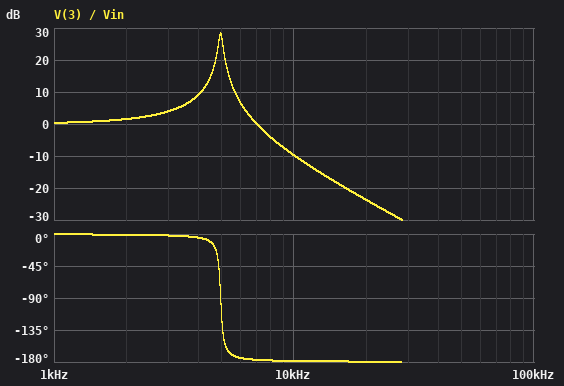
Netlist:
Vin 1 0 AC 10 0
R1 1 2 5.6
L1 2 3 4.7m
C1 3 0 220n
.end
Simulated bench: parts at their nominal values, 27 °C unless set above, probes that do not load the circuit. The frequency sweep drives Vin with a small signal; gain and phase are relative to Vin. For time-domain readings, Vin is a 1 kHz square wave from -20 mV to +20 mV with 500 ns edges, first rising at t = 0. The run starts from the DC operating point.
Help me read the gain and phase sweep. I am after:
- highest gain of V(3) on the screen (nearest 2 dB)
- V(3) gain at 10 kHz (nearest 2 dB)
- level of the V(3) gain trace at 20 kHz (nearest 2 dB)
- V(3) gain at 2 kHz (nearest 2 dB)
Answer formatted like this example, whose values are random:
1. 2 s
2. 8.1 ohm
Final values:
1. 28 dB
2. -10 dB
3. -24 dB
4. 2 dB
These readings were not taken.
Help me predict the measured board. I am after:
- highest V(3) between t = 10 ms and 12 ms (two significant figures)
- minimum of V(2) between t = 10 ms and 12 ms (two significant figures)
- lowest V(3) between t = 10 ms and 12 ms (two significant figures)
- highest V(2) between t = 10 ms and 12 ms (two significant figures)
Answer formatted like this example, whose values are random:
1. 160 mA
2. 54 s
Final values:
1. 150 mV
2. -25 mV
3. -150 mV
4. 25 mV
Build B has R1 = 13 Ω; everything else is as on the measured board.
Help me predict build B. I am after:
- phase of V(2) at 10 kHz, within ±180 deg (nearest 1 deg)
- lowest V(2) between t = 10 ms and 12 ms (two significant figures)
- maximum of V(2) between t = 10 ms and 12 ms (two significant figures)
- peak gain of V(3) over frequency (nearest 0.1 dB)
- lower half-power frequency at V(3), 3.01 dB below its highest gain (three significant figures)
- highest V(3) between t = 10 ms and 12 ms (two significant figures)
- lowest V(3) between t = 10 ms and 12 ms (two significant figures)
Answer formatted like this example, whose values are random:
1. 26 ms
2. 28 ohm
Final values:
1. 3 deg
2. -26 mV
3. 26 mV
4. 21.0 dB
5. 4.71 kHz
6. 87 mV
7. -87 mV
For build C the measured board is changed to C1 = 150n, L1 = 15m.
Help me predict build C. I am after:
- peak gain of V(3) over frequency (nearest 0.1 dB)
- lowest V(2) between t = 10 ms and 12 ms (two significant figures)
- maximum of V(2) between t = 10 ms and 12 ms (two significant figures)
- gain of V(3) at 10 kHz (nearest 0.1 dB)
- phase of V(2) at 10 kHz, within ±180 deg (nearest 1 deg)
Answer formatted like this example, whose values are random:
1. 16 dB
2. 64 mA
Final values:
1. 35.0 dB
2. -21 mV
3. 21 mV
4. -17.9 dB
5. 0 deg
